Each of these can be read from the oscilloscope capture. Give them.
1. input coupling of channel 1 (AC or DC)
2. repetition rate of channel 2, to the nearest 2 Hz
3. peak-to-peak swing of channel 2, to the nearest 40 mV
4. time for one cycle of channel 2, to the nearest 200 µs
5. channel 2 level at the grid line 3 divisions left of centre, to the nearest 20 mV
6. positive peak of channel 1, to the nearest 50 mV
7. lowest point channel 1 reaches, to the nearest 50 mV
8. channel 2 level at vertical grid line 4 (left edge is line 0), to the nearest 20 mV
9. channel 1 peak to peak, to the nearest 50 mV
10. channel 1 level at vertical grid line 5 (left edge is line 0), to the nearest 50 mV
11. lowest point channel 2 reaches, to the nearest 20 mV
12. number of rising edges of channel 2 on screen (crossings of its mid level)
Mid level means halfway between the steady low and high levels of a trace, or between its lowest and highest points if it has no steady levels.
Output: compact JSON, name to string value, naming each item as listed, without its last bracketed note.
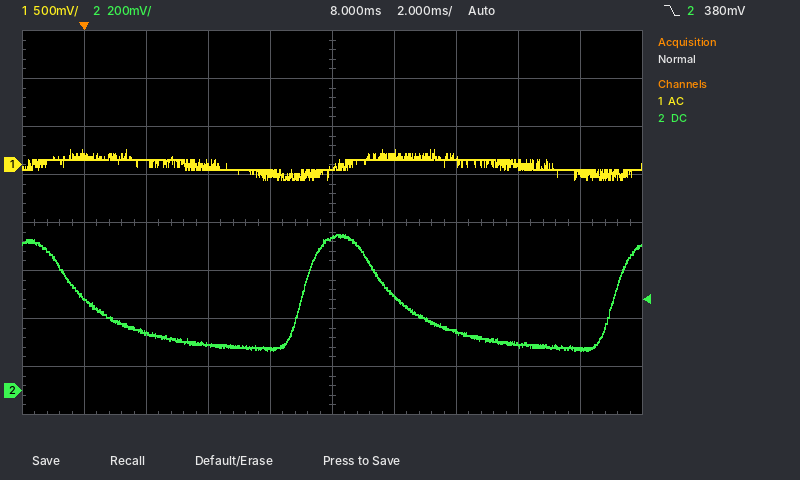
{"input coupling of channel 1": "AC", "repetition rate of channel 2, to the nearest 2 Hz": "100 Hz", "peak-to-peak swing of channel 2, to the nearest 40 mV": "480 mV", "time for one cycle of channel 2, to the nearest 200 µs": "10.0 ms", "channel 2 level at the grid line 3 divisions left of centre, to the nearest 20 mV": "240 mV", "positive peak of channel 1, to the nearest 50 mV": "150 mV", "lowest point channel 1 reaches, to the nearest 50 mV": "-150 mV", "channel 2 level at vertical grid line 4 (left edge is line 0), to the nearest 20 mV": "180 mV", "channel 1 peak to peak, to the nearest 50 mV": "300 mV", "channel 1 level at vertical grid line 5 (left edge is line 0), to the nearest 50 mV": "-50 mV", "lowest point channel 2 reaches, to the nearest 20 mV": "160 mV", "number of rising edges of channel 2 on screen": "2"}
